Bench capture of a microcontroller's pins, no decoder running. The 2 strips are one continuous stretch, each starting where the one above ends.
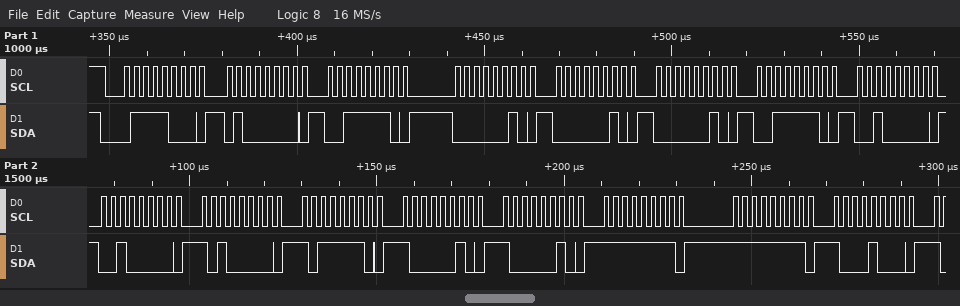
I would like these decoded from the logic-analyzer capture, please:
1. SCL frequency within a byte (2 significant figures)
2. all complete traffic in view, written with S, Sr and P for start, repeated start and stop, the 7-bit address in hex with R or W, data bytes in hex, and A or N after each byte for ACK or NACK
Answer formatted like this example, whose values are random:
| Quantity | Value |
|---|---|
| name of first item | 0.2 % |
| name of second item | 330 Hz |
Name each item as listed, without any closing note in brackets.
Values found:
| Quantity | Value |
|---|---|
| SCL frequency within a byte | 400 kHz |
| all complete traffic in view, written with S, Sr and P for start, repeated start and stop, the 7-bit address in hex with R or W, data bytes in hex, and A or N after each byte for ACK or NACK | S 3CW A 40 A 3E A 02 A 02 A 02 A 3E A 20 A 20 A A0 A BE A 82 A 82 A FF A FF A 88 A |
